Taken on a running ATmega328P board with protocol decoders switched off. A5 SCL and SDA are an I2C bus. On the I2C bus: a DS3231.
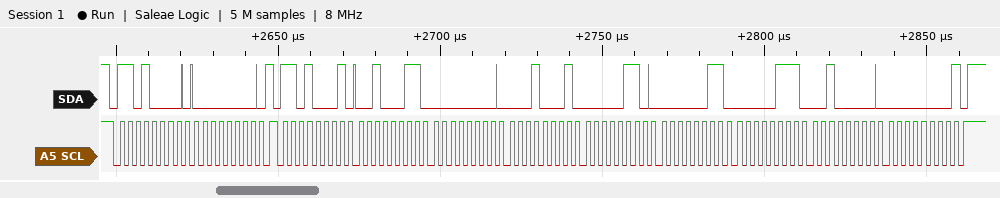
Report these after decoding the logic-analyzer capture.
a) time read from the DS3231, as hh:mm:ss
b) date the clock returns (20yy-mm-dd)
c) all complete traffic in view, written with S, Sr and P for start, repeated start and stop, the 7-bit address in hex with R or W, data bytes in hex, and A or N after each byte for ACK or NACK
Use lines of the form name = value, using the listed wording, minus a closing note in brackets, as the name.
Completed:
time read from the DS3231, as hh:mm:ss = 11:00:23
date the clock returns = 2020-07-03
all complete traffic in view, written with S, Sr and P for start, repeated start and stop, the 7-bit address in hex with R or W, data bytes in hex, and A or N after each byte for ACK or NACK = S 68W A 00 A Sr 68R A 23 A 00 A 11 A 06 A 03 A 07 A 20 A 00 N P
